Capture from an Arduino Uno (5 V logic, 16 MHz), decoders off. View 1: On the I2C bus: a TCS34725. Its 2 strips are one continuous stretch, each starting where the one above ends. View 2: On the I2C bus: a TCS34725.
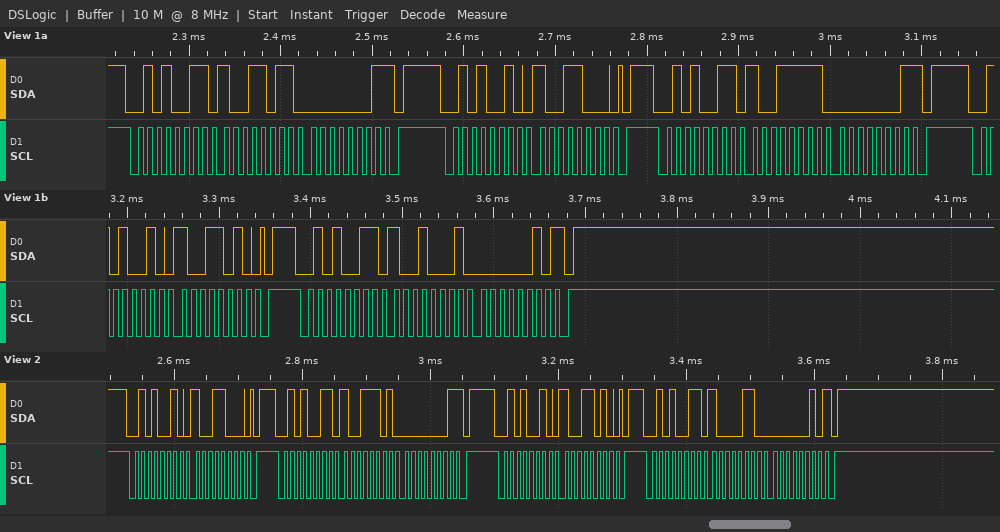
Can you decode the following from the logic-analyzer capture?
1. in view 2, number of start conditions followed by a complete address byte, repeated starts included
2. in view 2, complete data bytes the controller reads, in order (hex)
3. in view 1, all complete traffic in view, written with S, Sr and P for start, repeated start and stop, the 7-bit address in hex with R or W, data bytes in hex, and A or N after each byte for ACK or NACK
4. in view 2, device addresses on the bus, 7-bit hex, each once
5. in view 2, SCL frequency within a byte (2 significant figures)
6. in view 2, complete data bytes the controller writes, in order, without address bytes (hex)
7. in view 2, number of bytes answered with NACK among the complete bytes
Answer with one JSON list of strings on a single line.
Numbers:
["4", "9D 01 86 02", "S 29R A 9B A 01 N P S 29W A 98 A P S 29R A 9F A 01 N P S 29W A 9A A P S 29R A 91 A 02 N P", "0x29", "100 kHz", "98 9A", "2"]
